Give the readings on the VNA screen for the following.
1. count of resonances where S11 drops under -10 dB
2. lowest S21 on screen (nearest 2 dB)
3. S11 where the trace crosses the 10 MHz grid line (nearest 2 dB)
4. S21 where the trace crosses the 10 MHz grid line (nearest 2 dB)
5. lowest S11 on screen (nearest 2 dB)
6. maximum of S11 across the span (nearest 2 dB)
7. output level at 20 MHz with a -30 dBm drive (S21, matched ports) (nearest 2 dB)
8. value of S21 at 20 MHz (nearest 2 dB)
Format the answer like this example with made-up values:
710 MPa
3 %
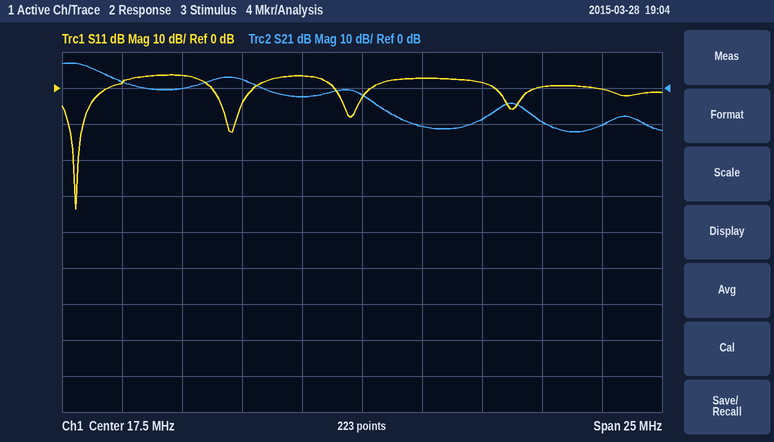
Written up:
2
-12 dB
4 dB
0 dB
-34 dB
4 dB
-40 dBm
-10 dB
